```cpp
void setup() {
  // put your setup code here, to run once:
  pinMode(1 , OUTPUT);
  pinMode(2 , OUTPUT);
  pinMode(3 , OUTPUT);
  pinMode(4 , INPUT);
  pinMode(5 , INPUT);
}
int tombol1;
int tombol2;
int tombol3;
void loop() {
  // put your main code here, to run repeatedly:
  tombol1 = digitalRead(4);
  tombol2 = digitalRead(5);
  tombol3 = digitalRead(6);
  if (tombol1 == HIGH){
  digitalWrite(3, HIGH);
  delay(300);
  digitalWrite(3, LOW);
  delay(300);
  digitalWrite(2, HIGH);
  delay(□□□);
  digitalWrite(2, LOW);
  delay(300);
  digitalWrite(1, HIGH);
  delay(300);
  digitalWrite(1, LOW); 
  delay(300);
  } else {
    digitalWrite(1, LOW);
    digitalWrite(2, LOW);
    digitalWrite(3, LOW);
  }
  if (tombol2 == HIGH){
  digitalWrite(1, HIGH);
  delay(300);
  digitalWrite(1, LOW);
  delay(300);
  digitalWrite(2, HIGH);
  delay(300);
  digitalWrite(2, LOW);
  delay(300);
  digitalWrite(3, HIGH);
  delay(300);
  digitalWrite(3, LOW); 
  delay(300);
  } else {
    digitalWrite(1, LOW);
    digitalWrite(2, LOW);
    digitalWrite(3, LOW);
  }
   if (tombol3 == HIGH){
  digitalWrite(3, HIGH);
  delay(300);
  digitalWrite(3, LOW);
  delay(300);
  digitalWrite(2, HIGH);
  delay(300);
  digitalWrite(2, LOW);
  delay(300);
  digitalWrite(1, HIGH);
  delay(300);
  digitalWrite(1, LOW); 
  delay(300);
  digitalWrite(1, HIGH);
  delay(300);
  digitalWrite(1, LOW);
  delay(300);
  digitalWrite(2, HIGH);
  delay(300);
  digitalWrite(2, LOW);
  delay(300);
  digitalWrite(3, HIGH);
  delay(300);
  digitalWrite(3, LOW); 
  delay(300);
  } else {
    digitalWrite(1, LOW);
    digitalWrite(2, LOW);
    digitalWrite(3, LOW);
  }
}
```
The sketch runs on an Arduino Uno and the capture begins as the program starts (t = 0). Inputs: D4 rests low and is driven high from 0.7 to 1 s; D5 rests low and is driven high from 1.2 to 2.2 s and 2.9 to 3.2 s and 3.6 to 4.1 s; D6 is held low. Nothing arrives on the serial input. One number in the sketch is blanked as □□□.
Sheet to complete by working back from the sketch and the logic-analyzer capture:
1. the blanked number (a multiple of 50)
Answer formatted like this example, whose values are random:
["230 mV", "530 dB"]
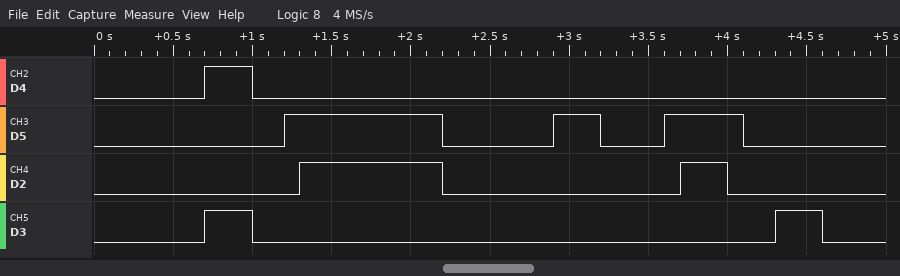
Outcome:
["900"]
